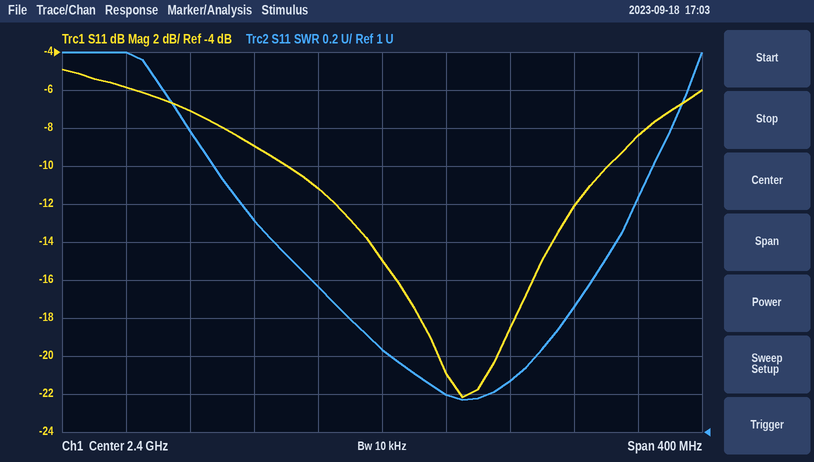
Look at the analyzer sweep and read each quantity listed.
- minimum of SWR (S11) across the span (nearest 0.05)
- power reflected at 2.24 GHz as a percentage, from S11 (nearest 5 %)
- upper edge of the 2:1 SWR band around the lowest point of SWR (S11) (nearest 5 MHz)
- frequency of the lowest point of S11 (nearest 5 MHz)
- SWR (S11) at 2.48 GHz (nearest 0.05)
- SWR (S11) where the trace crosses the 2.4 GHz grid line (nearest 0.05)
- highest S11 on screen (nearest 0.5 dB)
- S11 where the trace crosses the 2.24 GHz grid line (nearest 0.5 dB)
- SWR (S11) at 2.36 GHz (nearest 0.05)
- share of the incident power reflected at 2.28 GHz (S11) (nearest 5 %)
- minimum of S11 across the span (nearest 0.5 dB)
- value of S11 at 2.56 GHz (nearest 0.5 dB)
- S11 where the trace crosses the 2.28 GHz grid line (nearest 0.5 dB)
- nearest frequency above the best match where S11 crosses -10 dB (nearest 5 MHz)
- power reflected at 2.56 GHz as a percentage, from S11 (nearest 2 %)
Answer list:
1.15
25 %
2.545 GHz
2.450 GHz
1.25
1.45
-5.0 dB
-6.0 dB
1.75
20 %
-22.0 dB
-8.5 dB
-7.0 dB
2.540 GHz
14 %
